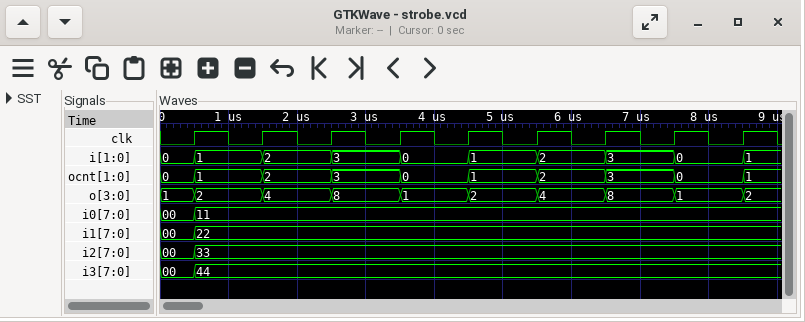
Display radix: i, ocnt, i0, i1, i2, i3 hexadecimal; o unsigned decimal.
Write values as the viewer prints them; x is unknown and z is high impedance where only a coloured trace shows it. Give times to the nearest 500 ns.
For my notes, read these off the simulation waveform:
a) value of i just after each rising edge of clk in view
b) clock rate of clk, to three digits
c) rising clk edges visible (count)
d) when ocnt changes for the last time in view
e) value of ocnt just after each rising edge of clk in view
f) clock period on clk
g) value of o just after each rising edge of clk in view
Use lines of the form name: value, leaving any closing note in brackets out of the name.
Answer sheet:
value of i just after each rising edge of clk in view: 1, 2, 3, 0, 1, 2, 3, 0, 1
clock rate of clk, to three digits: 1.00 MHz
rising clk edges visible: 9
when ocnt changes for the last time in view: 8500 ns
value of ocnt just after each rising edge of clk in view: 1, 2, 3, 0, 1, 2, 3, 0, 1
clock period on clk: 1000 ns
value of o just after each rising edge of clk in view: 2, 4, 8, 1, 2, 4, 8, 1, 2
